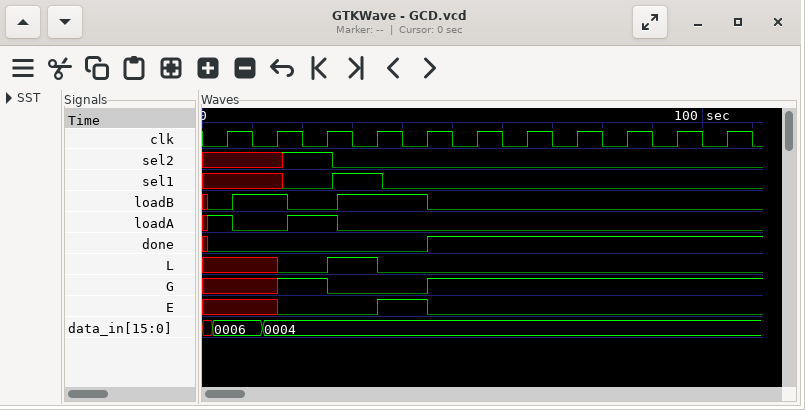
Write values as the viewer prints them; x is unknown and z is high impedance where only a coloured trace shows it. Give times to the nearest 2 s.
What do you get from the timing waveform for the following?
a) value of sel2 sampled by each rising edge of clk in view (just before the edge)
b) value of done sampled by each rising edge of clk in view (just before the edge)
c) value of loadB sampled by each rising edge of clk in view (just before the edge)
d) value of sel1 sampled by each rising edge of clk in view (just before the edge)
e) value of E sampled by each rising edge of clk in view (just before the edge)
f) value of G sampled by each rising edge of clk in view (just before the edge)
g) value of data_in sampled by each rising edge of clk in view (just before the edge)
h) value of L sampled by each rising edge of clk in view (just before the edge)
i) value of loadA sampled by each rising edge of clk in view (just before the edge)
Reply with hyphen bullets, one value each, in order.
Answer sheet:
- x x 1 0 0 0 0 0 0 0 0
- 0 0 0 0 0 1 1 1 1 1 1
- 0 1 0 1 1 0 0 0 0 0 0
- x x 0 1 0 0 0 0 0 0 0
- x x 0 0 1 0 0 0 0 0 0
- x x 1 0 0 1 1 1 1 1 1
- 0006, 0004, 0004, 0004, 0004, 0004, 0004, 0004, 0004, 0004, 0004
- x x 0 1 0 0 0 0 0 0 0
- 1 0 1 0 0 0 0 0 0 0 0
